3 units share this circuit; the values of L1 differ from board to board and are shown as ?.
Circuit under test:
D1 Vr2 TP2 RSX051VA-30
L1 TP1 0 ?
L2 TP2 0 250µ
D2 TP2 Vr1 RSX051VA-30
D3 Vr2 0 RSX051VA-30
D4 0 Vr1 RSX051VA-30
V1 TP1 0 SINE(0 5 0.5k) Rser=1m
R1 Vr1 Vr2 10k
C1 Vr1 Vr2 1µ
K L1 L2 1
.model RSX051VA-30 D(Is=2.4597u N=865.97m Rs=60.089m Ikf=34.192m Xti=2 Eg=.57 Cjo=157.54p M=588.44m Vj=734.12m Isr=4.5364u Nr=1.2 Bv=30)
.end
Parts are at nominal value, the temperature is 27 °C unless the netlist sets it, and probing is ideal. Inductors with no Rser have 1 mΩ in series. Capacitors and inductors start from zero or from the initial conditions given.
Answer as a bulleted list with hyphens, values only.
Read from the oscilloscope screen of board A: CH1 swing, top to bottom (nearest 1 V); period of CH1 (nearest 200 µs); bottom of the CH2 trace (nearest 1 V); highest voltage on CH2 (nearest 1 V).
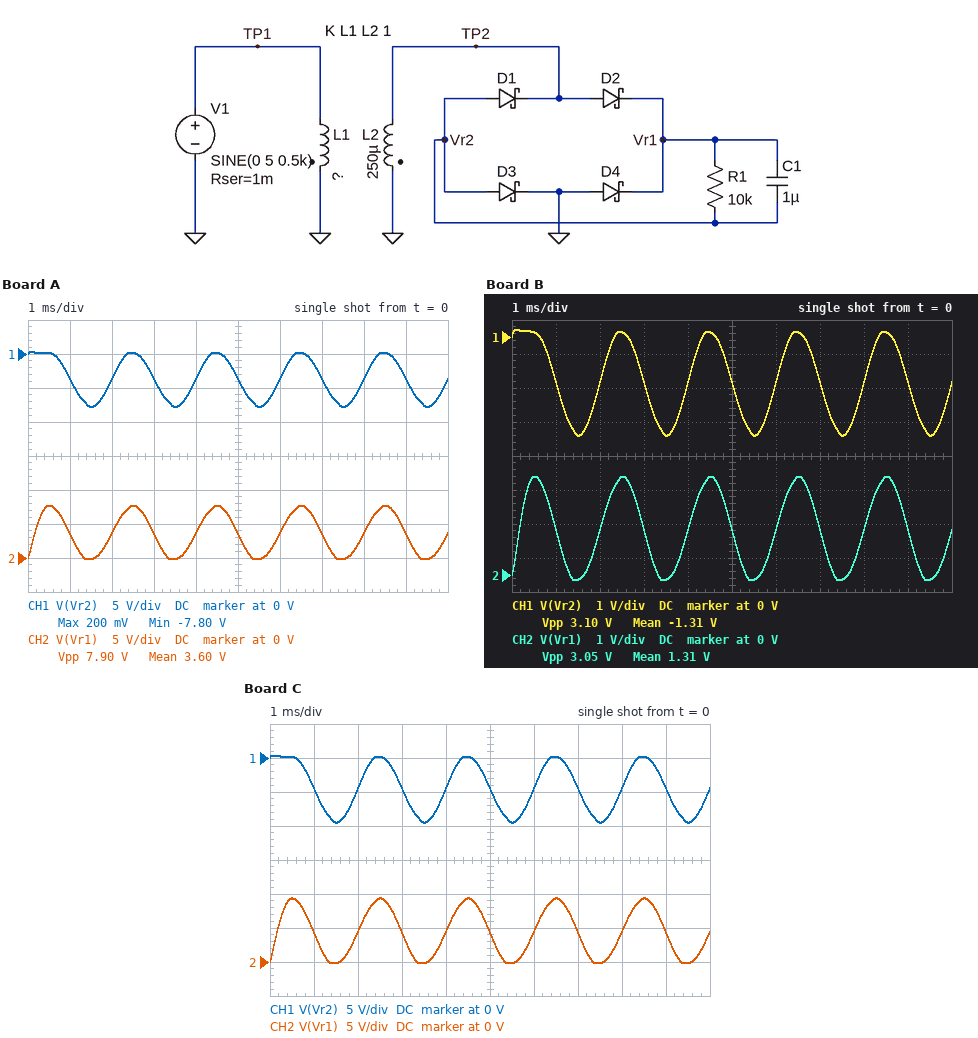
- 8 V
- 2.0 ms
- 0 V
- 8 V
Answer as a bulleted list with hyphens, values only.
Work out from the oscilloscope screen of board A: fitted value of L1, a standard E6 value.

- 100 µH
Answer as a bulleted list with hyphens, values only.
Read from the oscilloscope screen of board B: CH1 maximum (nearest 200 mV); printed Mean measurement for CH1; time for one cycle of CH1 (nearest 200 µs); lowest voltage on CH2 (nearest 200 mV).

- 200 mV
- -1.31 V
- 2.0 ms
- -200 mV
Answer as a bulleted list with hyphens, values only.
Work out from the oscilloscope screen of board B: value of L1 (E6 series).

- 680 µH
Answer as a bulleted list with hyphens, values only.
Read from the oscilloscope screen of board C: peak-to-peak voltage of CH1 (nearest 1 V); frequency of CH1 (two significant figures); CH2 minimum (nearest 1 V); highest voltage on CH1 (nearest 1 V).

- 10 V
- 500 Hz
- 0 V
- 0 V
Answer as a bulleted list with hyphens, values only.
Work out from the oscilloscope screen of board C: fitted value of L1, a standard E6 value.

- 68 µH
